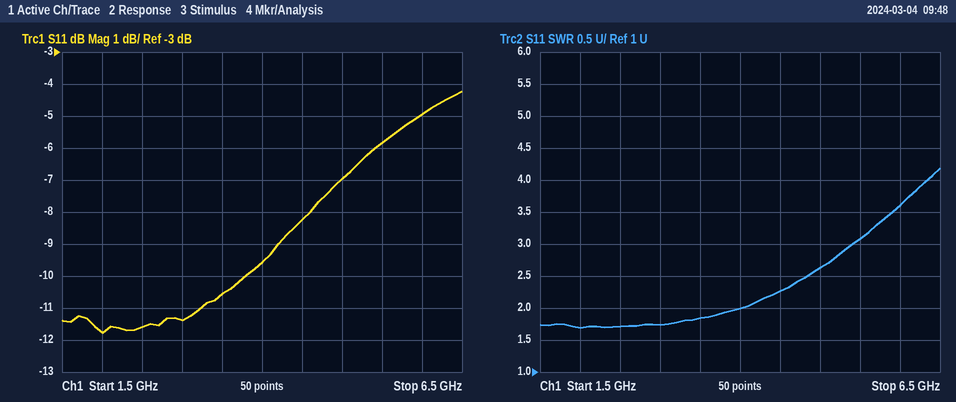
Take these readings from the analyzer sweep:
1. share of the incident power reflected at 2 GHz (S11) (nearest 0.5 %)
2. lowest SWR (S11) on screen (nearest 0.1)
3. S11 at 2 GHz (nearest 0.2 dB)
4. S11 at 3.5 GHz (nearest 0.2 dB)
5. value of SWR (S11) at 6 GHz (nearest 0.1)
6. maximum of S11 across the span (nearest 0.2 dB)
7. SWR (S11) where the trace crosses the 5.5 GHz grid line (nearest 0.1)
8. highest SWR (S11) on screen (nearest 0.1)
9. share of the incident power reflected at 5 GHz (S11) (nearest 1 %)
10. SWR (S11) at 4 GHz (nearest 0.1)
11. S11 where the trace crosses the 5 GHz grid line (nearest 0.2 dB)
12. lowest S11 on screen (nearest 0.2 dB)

6.5 %
1.7
-11.8 dB
-10.6 dB
3.6
-4.2 dB
3.1
4.2
20 %
2.0
-7.0 dB
-11.8 dB
